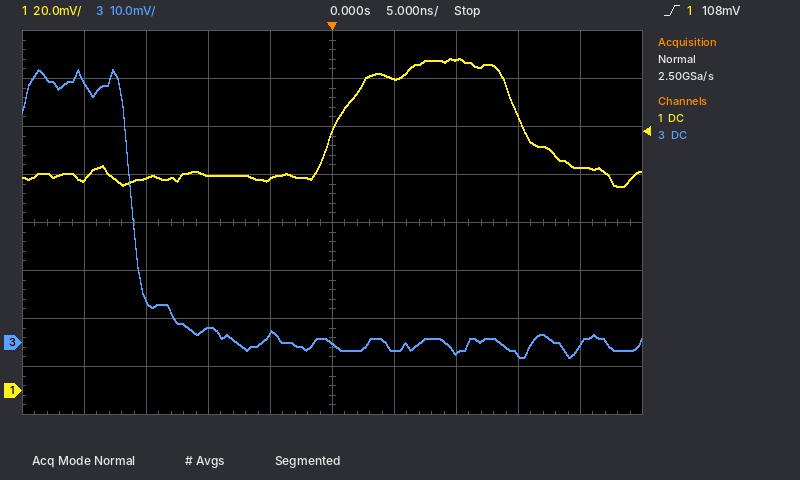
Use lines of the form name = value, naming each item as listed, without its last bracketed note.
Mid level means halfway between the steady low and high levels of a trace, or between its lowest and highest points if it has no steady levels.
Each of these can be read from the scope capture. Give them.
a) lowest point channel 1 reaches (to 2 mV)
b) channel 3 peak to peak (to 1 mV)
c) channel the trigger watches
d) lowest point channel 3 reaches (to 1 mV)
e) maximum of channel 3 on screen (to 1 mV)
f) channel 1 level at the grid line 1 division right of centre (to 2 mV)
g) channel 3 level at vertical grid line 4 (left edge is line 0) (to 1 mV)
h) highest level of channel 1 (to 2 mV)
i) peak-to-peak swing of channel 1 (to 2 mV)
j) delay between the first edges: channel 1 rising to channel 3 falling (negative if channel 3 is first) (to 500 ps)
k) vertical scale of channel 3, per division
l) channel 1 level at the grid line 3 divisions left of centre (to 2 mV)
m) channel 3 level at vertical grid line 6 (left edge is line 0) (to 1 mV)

lowest point channel 1 reaches = 84 mV
channel 3 peak to peak = 60 mV
channel the trigger watches = channel 1
lowest point channel 3 reaches = -3 mV
maximum of channel 3 on screen = 57 mV
channel 1 level at the grid line 1 division right of centre = 130 mV
channel 3 level at vertical grid line 4 (left edge is line 0) = 2 mV
highest level of channel 1 = 138 mV
peak-to-peak swing of channel 1 = 54 mV
delay between the first edges: channel 1 rising to channel 3 falling (negative if channel 3 is first) = -16.5 ns
vertical scale of channel 3, per division = 10 mV
channel 1 level at the grid line 3 divisions left of centre = 88 mV
channel 3 level at vertical grid line 6 (left edge is line 0) = -2 mV
